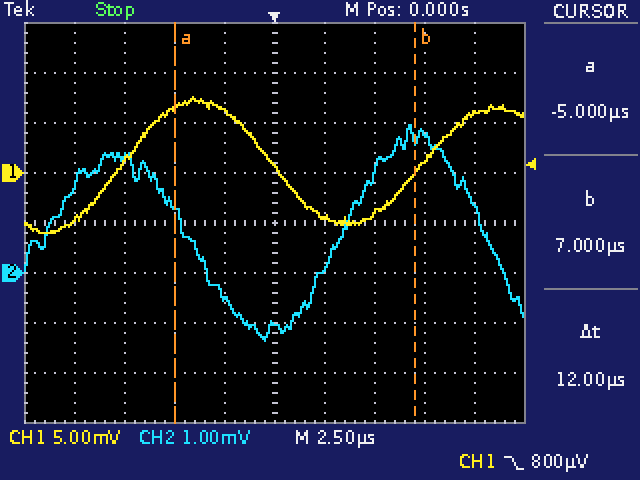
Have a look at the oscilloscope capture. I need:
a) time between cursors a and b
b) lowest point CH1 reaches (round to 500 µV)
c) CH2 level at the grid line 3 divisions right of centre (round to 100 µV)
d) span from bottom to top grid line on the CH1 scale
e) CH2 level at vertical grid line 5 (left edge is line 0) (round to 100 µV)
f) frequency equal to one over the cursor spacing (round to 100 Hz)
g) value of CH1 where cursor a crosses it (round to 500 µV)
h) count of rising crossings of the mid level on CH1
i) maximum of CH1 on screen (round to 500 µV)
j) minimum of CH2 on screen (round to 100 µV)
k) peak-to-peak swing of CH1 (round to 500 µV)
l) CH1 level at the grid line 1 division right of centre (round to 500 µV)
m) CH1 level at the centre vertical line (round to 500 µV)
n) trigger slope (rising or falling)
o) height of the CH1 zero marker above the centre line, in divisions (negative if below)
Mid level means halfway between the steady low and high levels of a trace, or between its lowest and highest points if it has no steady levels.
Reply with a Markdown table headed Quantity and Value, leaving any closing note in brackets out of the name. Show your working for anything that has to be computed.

| Quantity | Value |
|---|---|
| time between cursors a and b | 12 µs |
| lowest point CH1 reaches | -6.0 mV |
| CH2 level at the grid line 3 divisions right of centre | 2.8 mV |
| span from bottom to top grid line on the CH1 scale | 40 mV |
| CH2 level at vertical grid line 5 (left edge is line 0) | -1.0 mV |
| frequency equal to one over the cursor spacing | 1 / 12 µs ≈ 83.3 kHz |
| value of CH1 where cursor a crosses it | 6.5 mV |
| count of rising crossings of the mid level on CH1 | 2 |
| maximum of CH1 on screen | 7.5 mV |
| minimum of CH2 on screen | -1.4 mV |
| peak-to-peak swing of CH1 | 7.5 mV − (-6.0 mV) = 13.5 mV |
| CH1 level at the grid line 1 division right of centre | -4.5 mV |
| CH1 level at the centre vertical line | 500 µV |
| trigger slope | falling |
| height of the CH1 zero marker above the centre line, in divisions | +1.0 div |
